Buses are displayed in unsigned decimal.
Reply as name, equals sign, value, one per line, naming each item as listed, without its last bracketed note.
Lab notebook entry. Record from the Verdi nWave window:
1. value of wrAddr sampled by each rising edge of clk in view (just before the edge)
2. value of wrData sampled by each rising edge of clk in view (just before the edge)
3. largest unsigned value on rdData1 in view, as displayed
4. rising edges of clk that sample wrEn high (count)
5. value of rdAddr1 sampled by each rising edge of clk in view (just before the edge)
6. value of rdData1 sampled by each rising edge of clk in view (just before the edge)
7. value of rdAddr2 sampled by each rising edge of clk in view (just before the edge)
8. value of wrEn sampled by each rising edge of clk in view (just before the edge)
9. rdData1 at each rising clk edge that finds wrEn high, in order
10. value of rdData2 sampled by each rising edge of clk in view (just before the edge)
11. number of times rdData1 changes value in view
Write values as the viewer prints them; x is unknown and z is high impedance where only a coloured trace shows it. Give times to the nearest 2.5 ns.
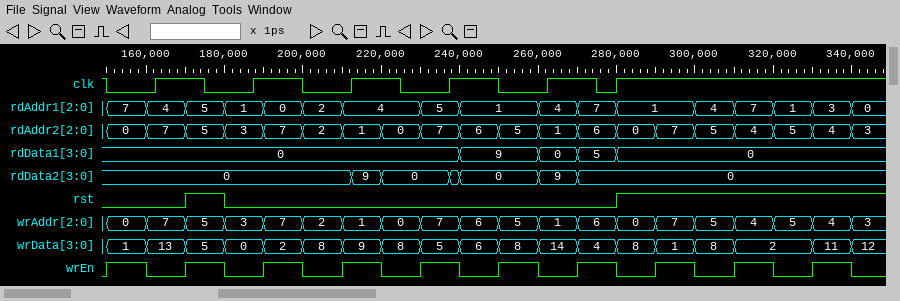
value of wrAddr sampled by each rising edge of clk in view = 7, 3, 1, 7, 1, 6
value of wrData sampled by each rising edge of clk in view = 13, 0, 9, 5, 14, 4
largest unsigned value on rdData1 in view, as displayed = 9
rising edges of clk that sample wrEn high = 3
value of rdAddr1 sampled by each rising edge of clk in view = 4, 1, 4, 5, 4, 7
value of rdData1 sampled by each rising edge of clk in view = 0, 0, 0, 0, 0, 5
value of rdAddr2 sampled by each rising edge of clk in view = 7, 3, 1, 7, 1, 6
value of wrEn sampled by each rising edge of clk in view = 0 0 1 1 0 1
rdData1 at each rising clk edge that finds wrEn high, in order = 0, 0, 5
value of rdData2 sampled by each rising edge of clk in view = 0, 0, 0, 0, 9, 0
number of times rdData1 changes value in view = 4
